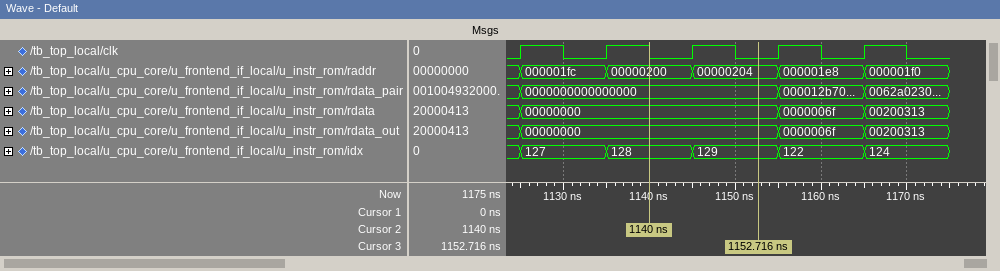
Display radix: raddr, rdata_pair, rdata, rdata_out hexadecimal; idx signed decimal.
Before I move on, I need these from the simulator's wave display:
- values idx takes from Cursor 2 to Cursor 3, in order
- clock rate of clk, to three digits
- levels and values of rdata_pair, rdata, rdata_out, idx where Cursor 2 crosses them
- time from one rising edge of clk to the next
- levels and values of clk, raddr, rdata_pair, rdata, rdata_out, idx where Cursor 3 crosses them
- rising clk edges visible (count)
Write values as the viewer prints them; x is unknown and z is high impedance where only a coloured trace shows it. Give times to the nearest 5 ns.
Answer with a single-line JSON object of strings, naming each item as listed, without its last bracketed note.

{"values idx takes from Cursor 2 to Cursor 3, in order": "128, 129", "clock rate of clk, to three digits": "100 MHz", "levels and values of rdata_pair, rdata, rdata_out, idx where Cursor 2 crosses them": "rdata_pair=0000000000000000, rdata=00000000, rdata_out=00000000, idx=128", "time from one rising edge of clk to the next": "10 ns", "levels and values of clk, raddr, rdata_pair, rdata, rdata_out, idx where Cursor 3 crosses them": "clk=0, raddr=00000204, rdata_pair=0000000000000000, rdata=00000000, rdata_out=00000000, idx=129", "rising clk edges visible": "5"}
